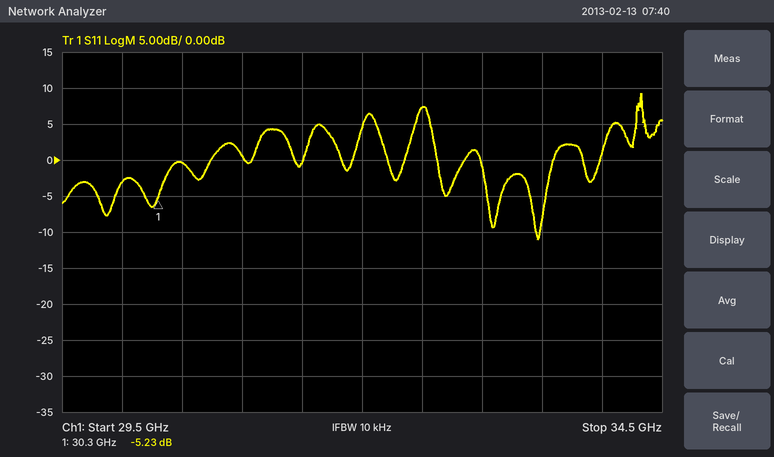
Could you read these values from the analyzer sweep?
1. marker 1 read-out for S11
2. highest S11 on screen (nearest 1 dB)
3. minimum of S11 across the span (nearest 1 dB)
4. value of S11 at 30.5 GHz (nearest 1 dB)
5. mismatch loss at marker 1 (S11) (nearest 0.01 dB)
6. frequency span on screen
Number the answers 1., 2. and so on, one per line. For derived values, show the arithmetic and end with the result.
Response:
1. -5.23 dB
2. 9 dB
3. -11 dB
4. 0 dB
5. −10 log10(1 − 10^(-5.23/10)) ≈ 1.55 dB
6. 5 GHz
